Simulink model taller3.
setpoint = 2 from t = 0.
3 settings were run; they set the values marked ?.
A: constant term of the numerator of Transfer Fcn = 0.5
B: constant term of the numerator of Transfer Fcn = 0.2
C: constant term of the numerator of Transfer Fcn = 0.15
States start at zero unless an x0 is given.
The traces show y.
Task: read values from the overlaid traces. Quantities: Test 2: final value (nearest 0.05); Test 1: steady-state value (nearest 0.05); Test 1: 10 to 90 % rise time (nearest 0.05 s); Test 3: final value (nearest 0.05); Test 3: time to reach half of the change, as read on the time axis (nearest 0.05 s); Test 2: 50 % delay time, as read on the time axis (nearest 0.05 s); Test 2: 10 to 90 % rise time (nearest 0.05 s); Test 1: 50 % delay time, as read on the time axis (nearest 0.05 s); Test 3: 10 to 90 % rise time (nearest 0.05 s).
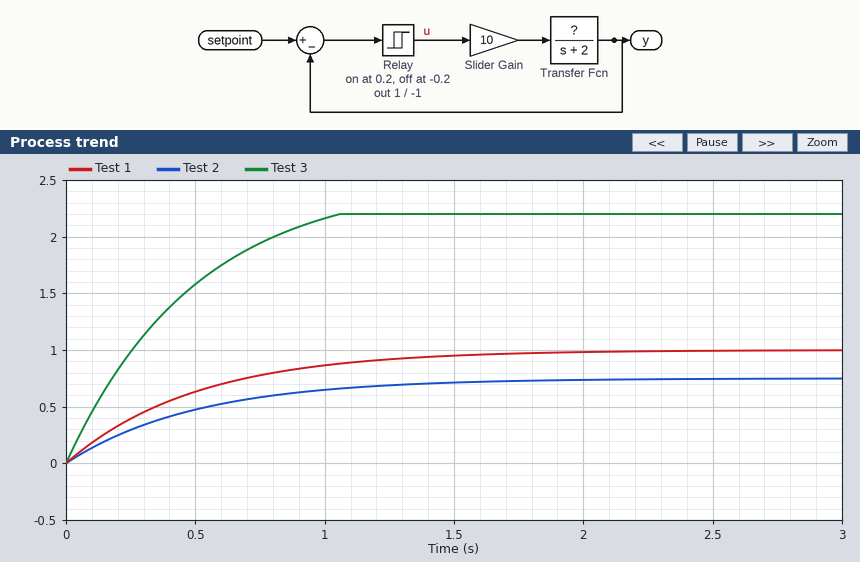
0.75
1.00
1.10 s
2.20
0.30 s
0.35 s
1.10 s
0.35 s
0.75 s
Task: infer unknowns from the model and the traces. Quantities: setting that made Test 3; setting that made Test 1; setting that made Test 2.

A
B
C
